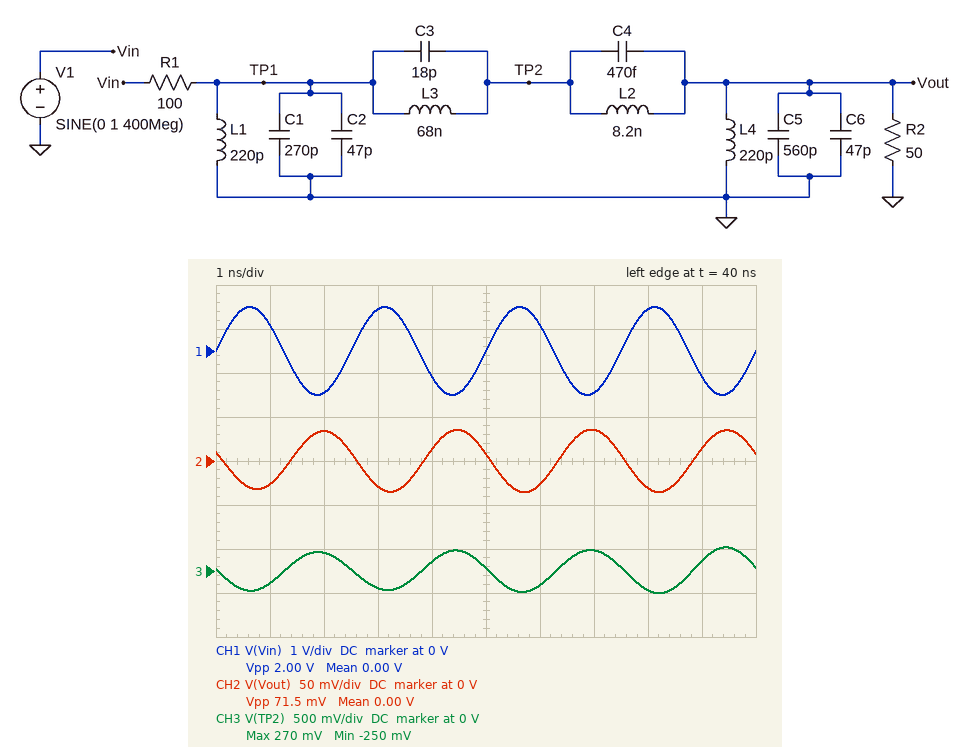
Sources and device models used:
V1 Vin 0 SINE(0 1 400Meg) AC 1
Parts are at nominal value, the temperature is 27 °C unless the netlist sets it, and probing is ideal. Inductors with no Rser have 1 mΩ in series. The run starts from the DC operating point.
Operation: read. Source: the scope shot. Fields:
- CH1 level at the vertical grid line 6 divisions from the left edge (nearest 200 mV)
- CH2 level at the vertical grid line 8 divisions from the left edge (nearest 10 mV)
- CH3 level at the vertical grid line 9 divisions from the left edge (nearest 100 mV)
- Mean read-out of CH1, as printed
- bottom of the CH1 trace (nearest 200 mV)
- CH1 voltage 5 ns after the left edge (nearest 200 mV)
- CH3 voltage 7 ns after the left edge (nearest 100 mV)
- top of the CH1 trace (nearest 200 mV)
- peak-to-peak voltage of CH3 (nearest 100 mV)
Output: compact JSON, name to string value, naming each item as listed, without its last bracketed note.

{"CH1 level at the vertical grid line 6 divisions from the left edge": "600 mV", "CH2 level at the vertical grid line 8 divisions from the left edge": "-30 mV", "CH3 level at the vertical grid line 9 divisions from the left edge": "100 mV", "Mean read-out of CH1, as printed": "0.00 V", "bottom of the CH1 trace": "-1.0 V", "CH1 voltage 5 ns after the left edge": "0 V", "CH3 voltage 7 ns after the left edge": "200 mV", "top of the CH1 trace": "1.0 V", "peak-to-peak voltage of CH3": "500 mV"}
